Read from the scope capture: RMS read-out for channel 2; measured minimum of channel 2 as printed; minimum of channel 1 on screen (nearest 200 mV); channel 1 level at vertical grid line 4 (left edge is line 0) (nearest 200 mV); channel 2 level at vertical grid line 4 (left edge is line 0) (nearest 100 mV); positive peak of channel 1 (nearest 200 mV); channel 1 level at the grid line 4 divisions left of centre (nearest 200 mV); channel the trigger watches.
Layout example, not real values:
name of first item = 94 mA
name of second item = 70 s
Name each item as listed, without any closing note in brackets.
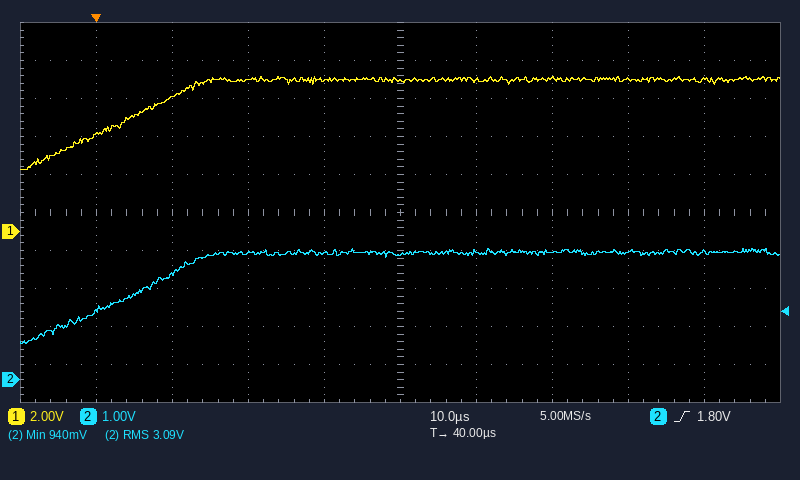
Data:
RMS read-out for channel 2 = 3.09 V
measured minimum of channel 2 as printed = 940 mV
minimum of channel 1 on screen = 3.2 V
channel 1 level at vertical grid line 4 (left edge is line 0) = 8.0 V
channel 2 level at vertical grid line 4 (left edge is line 0) = 3.3 V
positive peak of channel 1 = 8.2 V
channel 1 level at the grid line 4 divisions left of centre = 5.0 V
channel the trigger watches = channel 2
